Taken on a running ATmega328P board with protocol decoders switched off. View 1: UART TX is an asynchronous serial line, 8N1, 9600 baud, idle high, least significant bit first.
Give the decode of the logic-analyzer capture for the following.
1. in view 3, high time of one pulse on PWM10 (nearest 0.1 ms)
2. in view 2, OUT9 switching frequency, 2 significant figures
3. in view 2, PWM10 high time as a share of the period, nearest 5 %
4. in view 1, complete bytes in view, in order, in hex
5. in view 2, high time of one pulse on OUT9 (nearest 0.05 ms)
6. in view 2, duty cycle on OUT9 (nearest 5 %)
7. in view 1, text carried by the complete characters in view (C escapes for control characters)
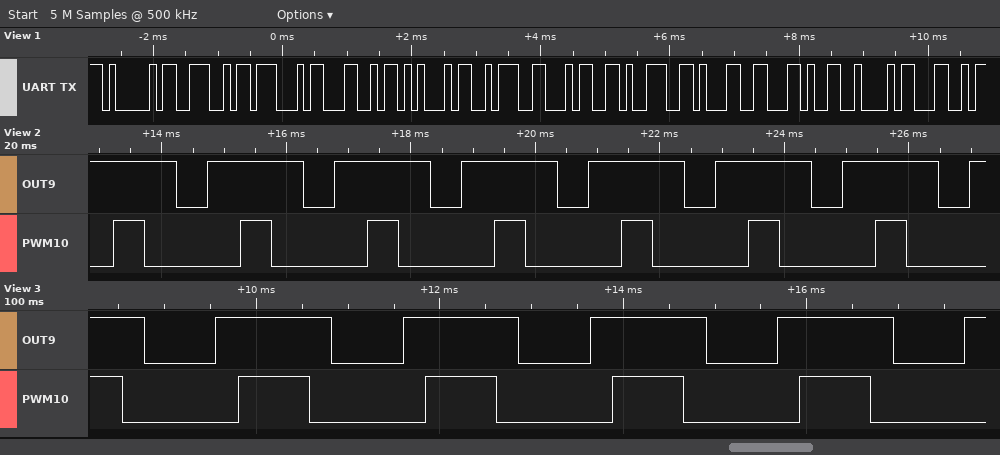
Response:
0.8 ms
490 Hz
25 %
41 4E 47 4C 45 3A 34 39 31 2C 42 4C
1.55 ms
75 %
"ANGLE:491,BL"
